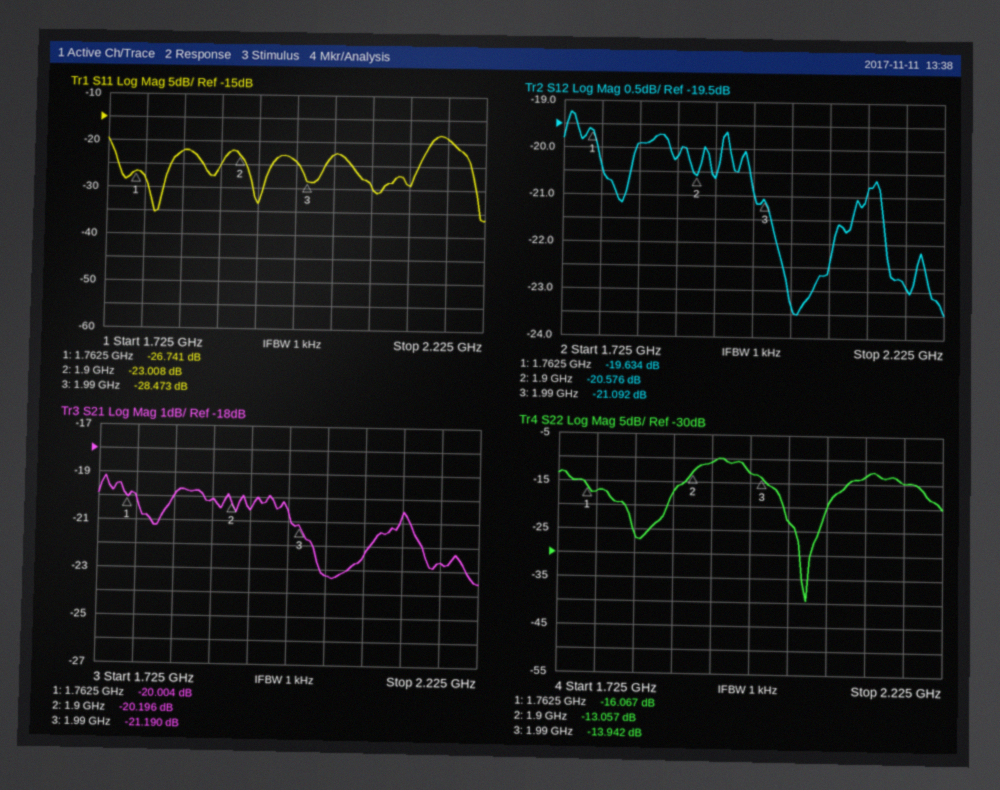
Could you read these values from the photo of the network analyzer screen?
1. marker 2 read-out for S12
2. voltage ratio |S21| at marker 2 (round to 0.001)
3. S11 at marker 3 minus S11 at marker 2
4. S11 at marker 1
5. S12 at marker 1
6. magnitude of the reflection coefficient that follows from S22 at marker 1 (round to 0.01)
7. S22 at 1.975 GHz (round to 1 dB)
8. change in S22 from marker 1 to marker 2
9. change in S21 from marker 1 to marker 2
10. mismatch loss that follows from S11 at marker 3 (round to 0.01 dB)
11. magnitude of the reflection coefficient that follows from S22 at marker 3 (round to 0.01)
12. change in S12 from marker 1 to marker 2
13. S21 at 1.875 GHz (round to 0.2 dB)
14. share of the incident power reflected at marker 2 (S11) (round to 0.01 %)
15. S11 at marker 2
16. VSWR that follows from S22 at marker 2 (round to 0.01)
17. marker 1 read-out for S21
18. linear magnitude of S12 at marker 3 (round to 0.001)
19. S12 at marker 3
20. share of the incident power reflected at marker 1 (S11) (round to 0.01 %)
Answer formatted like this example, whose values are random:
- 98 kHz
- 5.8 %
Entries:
- -20.576 dB
- 0.098
- -5.465 dB
- -26.741 dB
- -19.634 dB
- 0.16
- -13 dB
- 3.010 dB
- -0.192 dB
- 0.01 dB
- 0.20
- -0.942 dB
- -20.2 dB
- 0.50 %
- -23.008 dB
- 1.57
- -20.004 dB
- 0.088
- -21.092 dB
- 0.21 %
